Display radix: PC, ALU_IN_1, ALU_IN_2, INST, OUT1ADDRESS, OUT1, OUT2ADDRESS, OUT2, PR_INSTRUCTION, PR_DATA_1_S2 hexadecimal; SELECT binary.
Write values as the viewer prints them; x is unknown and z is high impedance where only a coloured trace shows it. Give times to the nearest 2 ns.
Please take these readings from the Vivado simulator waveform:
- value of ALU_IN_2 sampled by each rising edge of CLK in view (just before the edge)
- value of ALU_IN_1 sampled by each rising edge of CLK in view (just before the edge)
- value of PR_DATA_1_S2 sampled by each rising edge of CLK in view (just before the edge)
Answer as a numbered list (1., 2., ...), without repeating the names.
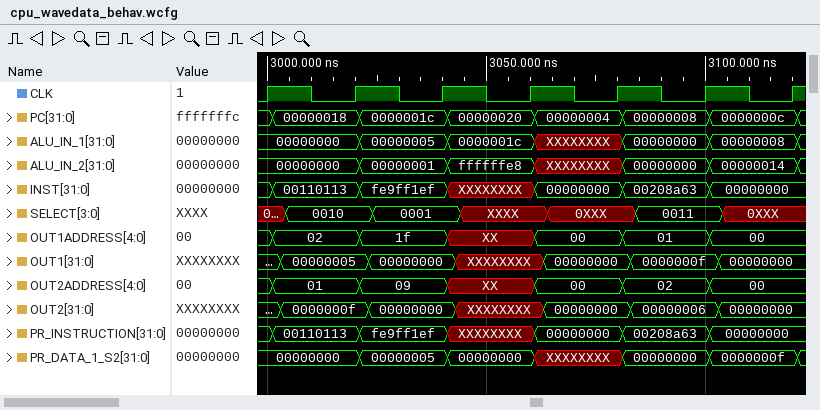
1. 00000000, 00000000, 00000001, ffffffe8, XXXXXXXX, 00000000, 00000014
2. 00000000, 00000000, 00000005, 0000001c, XXXXXXXX, 00000000, 00000008
3. 00000000, 00000000, 00000005, 00000000, XXXXXXXX, 00000000, 0000000f
